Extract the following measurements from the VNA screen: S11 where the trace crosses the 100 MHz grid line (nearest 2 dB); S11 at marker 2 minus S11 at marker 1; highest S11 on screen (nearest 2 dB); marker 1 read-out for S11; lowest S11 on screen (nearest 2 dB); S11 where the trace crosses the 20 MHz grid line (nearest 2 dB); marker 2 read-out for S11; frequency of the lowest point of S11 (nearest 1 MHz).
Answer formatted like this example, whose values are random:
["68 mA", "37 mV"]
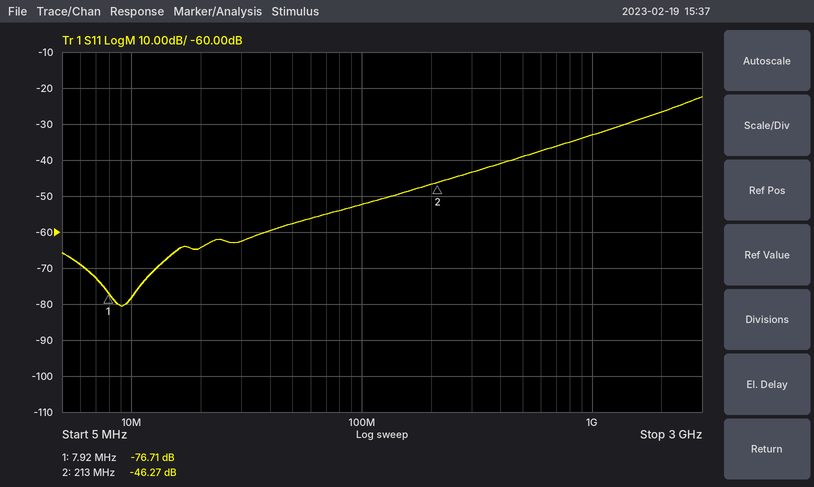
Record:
["-52 dB", "30.44 dB", "-22 dB", "-76.71 dB", "-80 dB", "-64 dB", "-46.27 dB", "9 MHz"]
